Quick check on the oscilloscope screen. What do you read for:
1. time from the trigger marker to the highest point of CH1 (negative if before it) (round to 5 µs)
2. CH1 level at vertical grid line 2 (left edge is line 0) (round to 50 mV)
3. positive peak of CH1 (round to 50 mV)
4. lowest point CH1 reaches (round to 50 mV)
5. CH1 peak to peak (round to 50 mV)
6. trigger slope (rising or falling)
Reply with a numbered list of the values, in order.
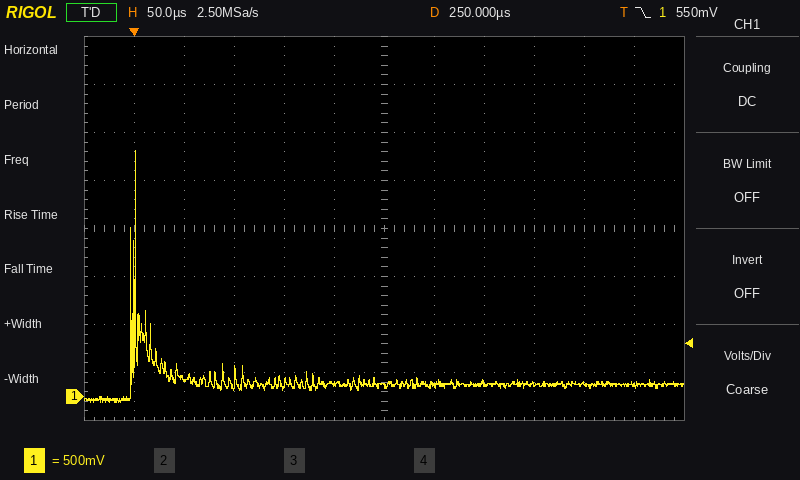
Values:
1. 0 µs
2. 200 mV
3. 2.55 V
4. -50 mV
5. 2.60 V
6. falling
